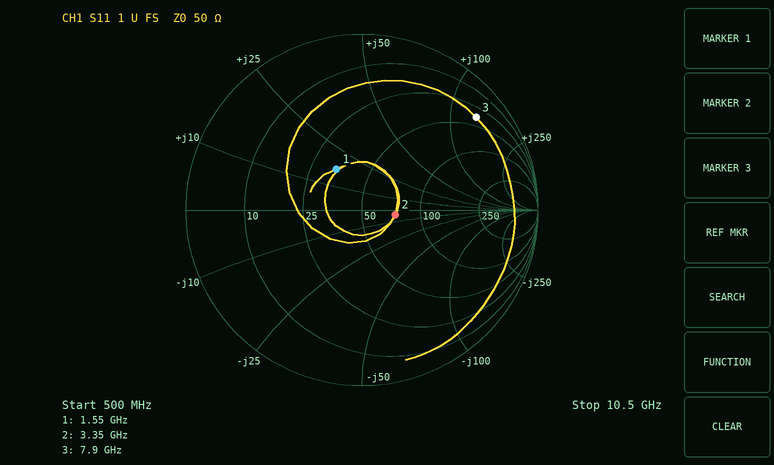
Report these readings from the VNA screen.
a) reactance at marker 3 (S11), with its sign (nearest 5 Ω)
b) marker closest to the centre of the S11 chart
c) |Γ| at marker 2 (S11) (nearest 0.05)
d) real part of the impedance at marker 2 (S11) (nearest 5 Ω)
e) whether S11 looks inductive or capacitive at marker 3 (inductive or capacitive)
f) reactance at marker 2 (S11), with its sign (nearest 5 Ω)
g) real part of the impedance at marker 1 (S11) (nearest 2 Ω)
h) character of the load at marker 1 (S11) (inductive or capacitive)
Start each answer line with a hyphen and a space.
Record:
- +130 Ω
- marker 2
- 0.20
- 75 Ω
- inductive
- -5 Ω
- 34 Ω
- inductive
